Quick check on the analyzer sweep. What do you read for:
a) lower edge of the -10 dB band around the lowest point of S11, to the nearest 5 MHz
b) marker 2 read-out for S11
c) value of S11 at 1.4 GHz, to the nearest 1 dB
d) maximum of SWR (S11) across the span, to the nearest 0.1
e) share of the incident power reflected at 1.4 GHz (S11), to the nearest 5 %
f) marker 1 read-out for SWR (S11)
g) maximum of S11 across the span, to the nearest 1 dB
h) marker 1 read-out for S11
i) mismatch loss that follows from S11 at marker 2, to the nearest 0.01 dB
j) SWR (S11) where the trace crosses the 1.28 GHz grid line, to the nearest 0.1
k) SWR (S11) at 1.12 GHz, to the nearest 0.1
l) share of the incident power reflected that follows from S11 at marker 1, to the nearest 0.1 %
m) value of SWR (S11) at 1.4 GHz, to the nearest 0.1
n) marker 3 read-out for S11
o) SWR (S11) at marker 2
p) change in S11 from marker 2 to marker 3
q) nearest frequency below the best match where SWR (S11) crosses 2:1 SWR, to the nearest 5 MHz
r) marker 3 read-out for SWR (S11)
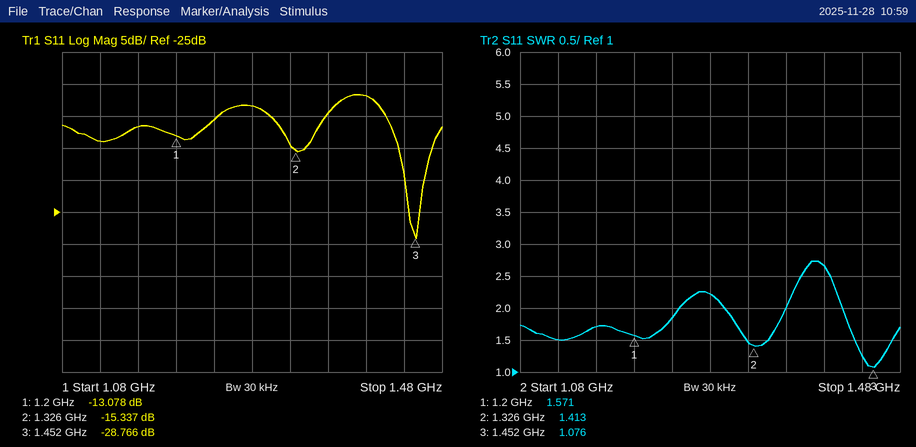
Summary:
1.420 GHz
-15.337 dB
-7 dB
2.7
20 %
1.571
-7 dB
-13.078 dB
0.13 dB
2.2
1.5
4.9 %
2.7
-28.766 dB
1.413
-13.429 dB
1.420 GHz
1.076
